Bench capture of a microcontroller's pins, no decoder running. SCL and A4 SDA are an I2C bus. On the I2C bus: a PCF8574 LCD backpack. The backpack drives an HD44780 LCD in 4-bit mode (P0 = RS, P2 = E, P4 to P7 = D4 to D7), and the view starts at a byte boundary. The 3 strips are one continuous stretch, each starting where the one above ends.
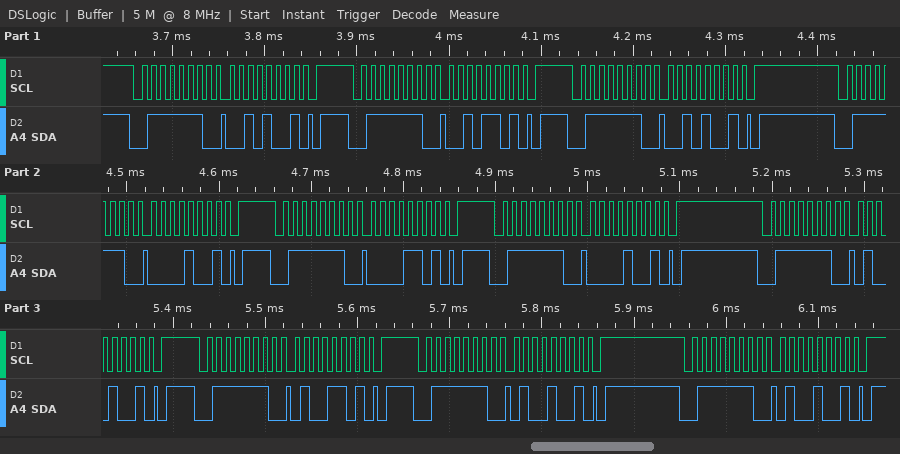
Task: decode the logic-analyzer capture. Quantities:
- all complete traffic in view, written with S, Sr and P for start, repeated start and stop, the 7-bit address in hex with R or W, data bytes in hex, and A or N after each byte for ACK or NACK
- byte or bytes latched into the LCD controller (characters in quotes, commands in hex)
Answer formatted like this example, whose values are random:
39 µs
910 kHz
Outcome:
S 3FW A 29 A P S 3FW A 2D A P S 3FW A 29 A P S 3FW A 09 A P S 3FW A 0D A P S 3FW A 09 A P S 3FW A 49 A P S 3FW A 4D A P S 3FW A 49 A P S 3FW A 49 A P
' '
